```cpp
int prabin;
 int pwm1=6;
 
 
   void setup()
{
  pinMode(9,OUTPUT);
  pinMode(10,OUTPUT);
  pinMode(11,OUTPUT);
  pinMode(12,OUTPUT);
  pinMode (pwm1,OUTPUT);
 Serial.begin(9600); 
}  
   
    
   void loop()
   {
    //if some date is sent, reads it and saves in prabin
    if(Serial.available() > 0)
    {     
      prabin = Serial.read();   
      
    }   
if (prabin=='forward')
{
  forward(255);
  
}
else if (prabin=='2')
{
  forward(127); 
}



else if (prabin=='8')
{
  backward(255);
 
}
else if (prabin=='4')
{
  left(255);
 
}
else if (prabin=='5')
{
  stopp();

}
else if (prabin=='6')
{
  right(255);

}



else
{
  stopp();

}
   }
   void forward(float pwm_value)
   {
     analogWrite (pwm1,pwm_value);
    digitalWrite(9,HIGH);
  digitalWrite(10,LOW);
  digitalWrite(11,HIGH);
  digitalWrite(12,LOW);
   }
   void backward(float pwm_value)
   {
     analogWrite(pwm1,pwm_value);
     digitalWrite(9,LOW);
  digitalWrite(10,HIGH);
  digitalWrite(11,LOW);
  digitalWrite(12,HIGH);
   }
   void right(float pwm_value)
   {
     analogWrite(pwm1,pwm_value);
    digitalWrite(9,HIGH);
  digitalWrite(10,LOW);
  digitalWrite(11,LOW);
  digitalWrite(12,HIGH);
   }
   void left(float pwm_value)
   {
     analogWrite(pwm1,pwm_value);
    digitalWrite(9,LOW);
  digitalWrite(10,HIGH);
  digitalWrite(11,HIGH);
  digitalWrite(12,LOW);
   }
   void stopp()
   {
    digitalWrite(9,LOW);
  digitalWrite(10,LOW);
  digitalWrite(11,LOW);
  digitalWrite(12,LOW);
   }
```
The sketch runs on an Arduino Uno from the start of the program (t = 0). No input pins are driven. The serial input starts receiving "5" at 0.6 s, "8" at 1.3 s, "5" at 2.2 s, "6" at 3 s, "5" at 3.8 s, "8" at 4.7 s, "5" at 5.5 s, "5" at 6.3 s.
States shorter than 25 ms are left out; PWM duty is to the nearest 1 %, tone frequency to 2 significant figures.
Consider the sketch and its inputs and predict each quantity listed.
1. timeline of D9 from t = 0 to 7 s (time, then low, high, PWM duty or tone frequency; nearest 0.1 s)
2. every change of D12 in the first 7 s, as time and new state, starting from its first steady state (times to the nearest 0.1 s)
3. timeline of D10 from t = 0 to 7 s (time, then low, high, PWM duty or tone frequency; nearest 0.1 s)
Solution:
0 s low; 3 s high; 3.8 s low
0 s low; 1.3 s high; 2.2 s low; 3 s high; 3.8 s low; 4.7 s high; 5.5 s low
0 s low; 1.3 s high; 2.2 s low; 4.7 s high; 5.5 s low
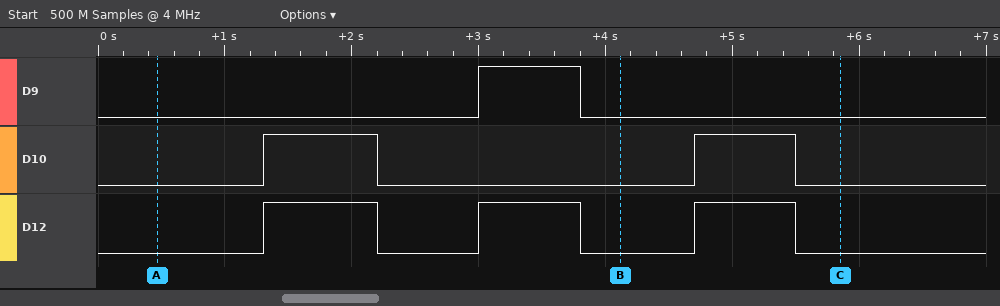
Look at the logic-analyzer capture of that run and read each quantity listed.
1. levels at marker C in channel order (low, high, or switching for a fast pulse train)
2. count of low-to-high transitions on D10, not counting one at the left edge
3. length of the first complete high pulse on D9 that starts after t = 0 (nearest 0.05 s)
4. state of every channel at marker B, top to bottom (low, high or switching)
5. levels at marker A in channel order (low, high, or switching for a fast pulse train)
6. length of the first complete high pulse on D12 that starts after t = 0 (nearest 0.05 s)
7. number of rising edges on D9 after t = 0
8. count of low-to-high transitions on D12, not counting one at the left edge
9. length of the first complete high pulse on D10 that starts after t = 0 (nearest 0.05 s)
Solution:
D9 low, D10 low, D12 low
2
0.80 s
D9 low, D10 low, D12 low
D9 low, D10 low, D12 low
0.90 s
1
3
0.90 s
